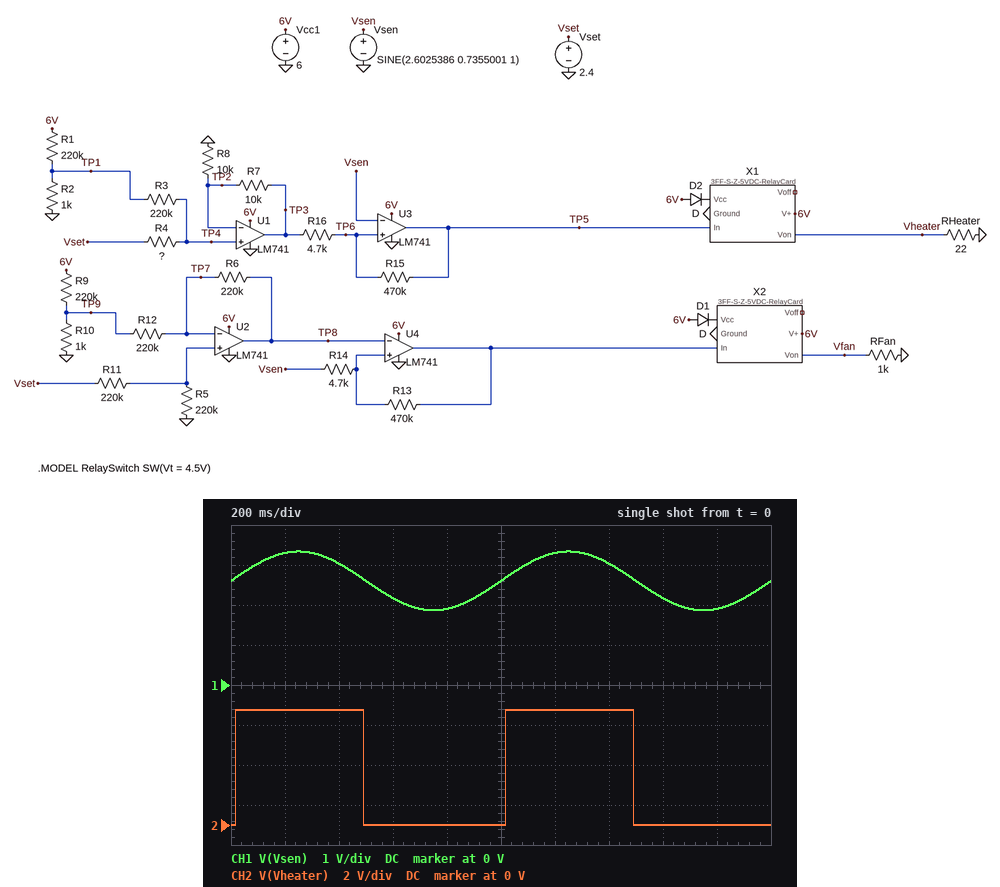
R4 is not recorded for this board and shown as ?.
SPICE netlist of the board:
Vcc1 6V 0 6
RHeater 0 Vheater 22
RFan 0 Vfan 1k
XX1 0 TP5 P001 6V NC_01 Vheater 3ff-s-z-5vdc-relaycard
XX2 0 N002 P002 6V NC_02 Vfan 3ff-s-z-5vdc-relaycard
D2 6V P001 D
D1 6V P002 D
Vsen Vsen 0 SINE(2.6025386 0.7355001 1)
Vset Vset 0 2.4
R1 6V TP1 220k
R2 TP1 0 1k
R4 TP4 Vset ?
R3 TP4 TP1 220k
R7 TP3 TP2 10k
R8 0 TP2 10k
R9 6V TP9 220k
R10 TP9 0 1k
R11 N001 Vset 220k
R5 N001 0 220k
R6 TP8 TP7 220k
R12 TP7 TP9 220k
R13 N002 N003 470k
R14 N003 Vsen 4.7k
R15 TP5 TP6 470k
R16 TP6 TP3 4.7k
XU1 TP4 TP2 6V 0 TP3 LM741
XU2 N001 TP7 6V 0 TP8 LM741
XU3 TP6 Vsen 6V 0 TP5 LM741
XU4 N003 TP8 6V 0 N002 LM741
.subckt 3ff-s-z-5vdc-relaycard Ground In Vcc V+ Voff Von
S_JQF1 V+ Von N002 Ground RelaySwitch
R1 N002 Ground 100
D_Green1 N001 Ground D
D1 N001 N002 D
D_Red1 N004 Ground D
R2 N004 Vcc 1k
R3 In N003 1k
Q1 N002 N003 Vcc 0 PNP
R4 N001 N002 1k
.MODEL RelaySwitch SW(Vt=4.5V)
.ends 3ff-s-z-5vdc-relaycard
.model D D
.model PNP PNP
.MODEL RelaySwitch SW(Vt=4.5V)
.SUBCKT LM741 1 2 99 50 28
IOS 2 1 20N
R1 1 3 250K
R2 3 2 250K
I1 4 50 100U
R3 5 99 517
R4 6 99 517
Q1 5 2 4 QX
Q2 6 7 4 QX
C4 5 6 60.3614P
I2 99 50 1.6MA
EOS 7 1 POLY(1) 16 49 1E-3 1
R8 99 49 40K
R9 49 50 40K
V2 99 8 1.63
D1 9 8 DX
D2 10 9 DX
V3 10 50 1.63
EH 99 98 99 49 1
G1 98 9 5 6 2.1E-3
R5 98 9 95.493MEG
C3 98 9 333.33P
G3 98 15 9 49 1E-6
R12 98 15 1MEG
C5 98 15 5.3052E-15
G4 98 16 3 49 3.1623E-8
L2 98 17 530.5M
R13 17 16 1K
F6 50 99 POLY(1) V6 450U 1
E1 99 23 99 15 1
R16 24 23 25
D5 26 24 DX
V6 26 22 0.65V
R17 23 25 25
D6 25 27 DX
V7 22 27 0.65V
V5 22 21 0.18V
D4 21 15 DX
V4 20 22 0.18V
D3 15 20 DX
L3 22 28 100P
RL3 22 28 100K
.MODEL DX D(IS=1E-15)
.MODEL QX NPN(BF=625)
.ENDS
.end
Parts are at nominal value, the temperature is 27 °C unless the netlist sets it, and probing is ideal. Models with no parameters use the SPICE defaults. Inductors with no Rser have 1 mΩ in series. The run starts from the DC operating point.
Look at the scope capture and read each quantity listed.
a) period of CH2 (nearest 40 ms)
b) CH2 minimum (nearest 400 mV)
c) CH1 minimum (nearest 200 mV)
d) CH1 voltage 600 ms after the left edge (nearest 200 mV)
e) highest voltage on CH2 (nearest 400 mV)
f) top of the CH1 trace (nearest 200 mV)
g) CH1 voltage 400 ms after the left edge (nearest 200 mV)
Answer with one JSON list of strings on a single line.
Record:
["1.00 s", "0 V", "1.8 V", "2.2 V", "5.6 V", "3.4 V", "3.0 V"]
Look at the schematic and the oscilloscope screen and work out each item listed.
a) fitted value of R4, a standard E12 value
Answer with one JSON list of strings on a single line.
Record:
["180 kΩ"]
